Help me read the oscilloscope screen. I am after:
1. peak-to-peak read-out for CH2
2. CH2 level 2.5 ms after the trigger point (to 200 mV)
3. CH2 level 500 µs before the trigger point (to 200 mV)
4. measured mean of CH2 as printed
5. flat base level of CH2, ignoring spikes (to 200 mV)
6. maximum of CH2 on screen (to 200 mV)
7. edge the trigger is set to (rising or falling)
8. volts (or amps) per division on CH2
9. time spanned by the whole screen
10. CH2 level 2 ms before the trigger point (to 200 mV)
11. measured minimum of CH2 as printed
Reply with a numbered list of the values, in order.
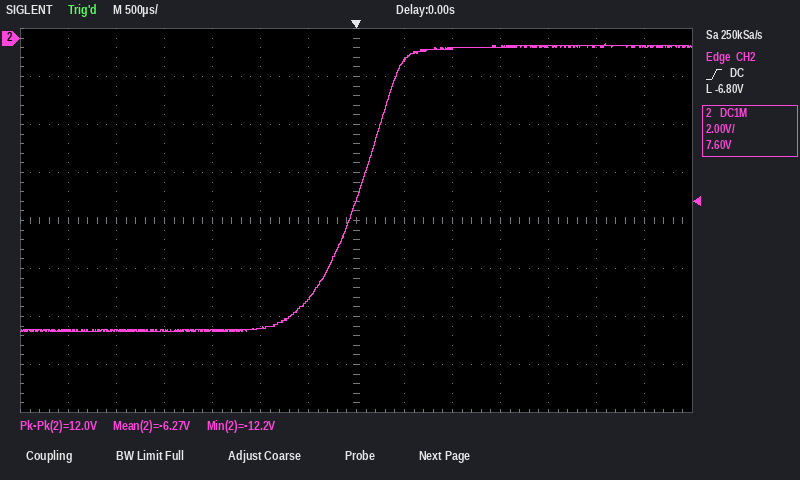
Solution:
1. 12.0 V
2. -400 mV
3. -10.8 V
4. -6.27 V
5. -12.2 V
6. -200 mV
7. rising
8. 2 V
9. 7 ms
10. -12.2 V
11. -12.2 V
